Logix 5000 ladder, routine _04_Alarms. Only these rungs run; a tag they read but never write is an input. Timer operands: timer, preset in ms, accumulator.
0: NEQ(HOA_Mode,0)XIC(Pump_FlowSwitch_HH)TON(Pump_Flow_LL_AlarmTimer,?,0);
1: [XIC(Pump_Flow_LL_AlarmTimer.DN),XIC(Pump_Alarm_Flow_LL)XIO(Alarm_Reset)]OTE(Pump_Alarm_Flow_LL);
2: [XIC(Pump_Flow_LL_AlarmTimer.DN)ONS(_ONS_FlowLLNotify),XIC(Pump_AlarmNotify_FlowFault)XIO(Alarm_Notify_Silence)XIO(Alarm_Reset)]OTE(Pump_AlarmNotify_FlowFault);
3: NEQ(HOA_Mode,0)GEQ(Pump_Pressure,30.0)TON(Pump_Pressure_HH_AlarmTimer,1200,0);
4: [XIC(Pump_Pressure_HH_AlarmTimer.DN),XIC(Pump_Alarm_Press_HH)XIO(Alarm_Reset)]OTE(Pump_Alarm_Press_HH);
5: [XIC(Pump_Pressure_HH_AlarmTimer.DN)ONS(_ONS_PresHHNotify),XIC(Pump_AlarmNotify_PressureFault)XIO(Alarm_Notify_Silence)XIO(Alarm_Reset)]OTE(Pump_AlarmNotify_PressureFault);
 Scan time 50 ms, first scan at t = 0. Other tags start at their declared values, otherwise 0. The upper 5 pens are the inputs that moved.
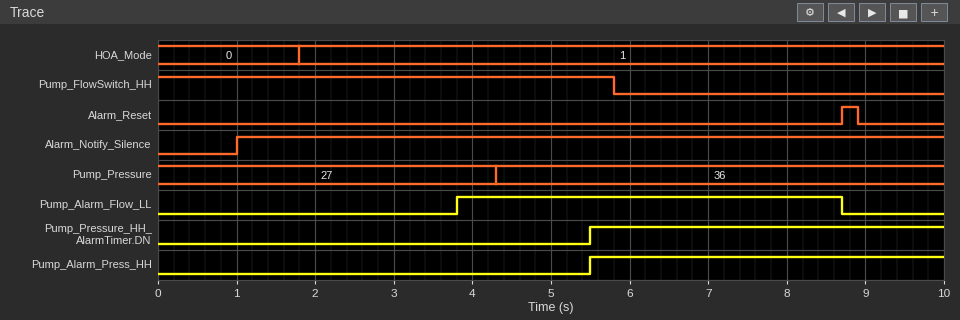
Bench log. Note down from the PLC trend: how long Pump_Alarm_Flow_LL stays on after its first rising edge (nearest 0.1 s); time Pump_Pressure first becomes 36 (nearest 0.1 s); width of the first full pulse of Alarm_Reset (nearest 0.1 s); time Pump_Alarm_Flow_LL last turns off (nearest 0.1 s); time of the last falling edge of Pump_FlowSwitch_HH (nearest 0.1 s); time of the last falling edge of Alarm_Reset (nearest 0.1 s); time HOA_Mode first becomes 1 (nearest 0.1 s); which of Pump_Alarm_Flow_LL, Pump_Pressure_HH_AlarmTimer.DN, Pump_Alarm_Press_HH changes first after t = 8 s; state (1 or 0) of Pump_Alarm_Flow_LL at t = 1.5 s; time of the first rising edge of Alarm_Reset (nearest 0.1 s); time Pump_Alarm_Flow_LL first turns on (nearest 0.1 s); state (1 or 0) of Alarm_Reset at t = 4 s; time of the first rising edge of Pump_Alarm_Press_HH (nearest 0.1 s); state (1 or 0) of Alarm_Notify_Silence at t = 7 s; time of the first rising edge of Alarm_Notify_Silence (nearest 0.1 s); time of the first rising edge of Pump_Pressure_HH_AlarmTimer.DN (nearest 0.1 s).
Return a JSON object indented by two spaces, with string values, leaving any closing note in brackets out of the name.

{
  "how long Pump_Alarm_Flow_LL stays on after its first rising edge": "4.9 s",
  "time Pump_Pressure first becomes 36": "4.3 s",
  "width of the first full pulse of Alarm_Reset": "0.2 s",
  "time Pump_Alarm_Flow_LL last turns off": "8.7 s",
  "time of the last falling edge of Pump_FlowSwitch_HH": "5.8 s",
  "time of the last falling edge of Alarm_Reset": "8.9 s",
  "time HOA_Mode first becomes 1": "1.8 s",
  "which of Pump_Alarm_Flow_LL, Pump_Pressure_HH_AlarmTimer.DN, Pump_Alarm_Press_HH changes first after t = 8 s": "Pump_Alarm_Flow_LL",
  "state (1 or 0) of Pump_Alarm_Flow_LL at t = 1.5 s": "0",
  "time of the first rising edge of Alarm_Reset": "8.7 s",
  "time Pump_Alarm_Flow_LL first turns on": "3.8 s",
  "state (1 or 0) of Alarm_Reset at t = 4 s": "0",
  "time of the first rising edge of Pump_Alarm_Press_HH": "5.5 s",
  "state (1 or 0) of Alarm_Notify_Silence at t = 7 s": "1",
  "time of the first rising edge of Alarm_Notify_Silence": "1.0 s",
  "time of the first rising edge of Pump_Pressure_HH_AlarmTimer.DN": "5.5 s"
}
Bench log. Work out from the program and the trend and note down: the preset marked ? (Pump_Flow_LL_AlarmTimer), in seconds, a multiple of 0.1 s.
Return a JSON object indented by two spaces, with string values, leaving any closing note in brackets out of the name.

{
  "the preset marked ? (Pump_Flow_LL_AlarmTimer), in seconds, a multiple of 0.1 s": "2.0 s"
}
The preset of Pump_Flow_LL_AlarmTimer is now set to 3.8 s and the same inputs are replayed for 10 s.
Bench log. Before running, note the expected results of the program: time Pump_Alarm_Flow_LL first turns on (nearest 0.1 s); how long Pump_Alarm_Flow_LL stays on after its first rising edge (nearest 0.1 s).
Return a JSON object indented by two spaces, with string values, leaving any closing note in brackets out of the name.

{
  "time Pump_Alarm_Flow_LL first turns on": "5.6 s",
  "how long Pump_Alarm_Flow_LL stays on after its first rising edge": "3.1 s"
}
